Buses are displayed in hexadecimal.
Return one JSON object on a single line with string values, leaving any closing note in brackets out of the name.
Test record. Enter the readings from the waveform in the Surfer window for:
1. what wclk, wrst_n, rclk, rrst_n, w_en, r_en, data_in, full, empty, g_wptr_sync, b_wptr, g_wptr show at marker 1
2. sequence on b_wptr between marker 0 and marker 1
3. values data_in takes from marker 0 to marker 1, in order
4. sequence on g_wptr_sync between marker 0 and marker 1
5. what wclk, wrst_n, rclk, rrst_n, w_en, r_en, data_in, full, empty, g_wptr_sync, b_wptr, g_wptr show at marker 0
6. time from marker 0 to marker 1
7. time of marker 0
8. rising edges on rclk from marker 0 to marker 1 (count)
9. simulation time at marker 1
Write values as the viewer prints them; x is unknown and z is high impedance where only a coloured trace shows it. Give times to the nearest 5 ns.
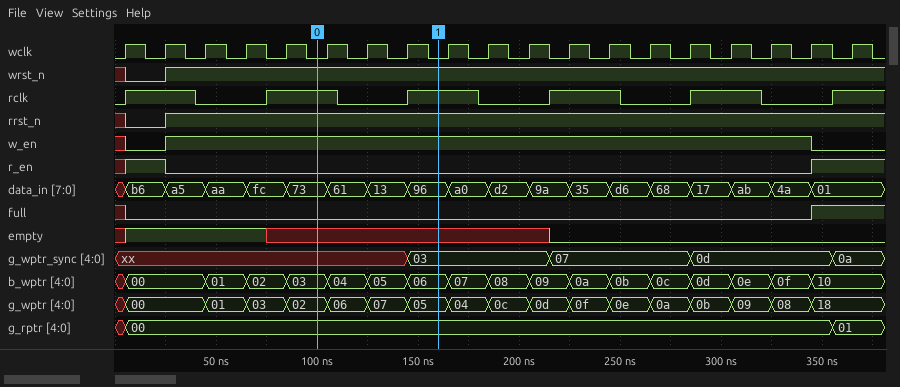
{"what wclk, wrst_n, rclk, rrst_n, w_en, r_en, data_in, full, empty, g_wptr_sync, b_wptr, g_wptr show at marker 1": "wclk=0, wrst_n=1, rclk=1, rrst_n=1, w_en=1, r_en=0, data_in=96, full=0, empty=x, g_wptr_sync=03, b_wptr=06, g_wptr=05", "sequence on b_wptr between marker 0 and marker 1": "03, 04, 05, 06", "values data_in takes from marker 0 to marker 1, in order": "73, 61, 13, 96", "sequence on g_wptr_sync between marker 0 and marker 1": "xx, 03", "what wclk, wrst_n, rclk, rrst_n, w_en, r_en, data_in, full, empty, g_wptr_sync, b_wptr, g_wptr show at marker 0": "wclk=0, wrst_n=1, rclk=1, rrst_n=1, w_en=1, r_en=0, data_in=73, full=0, empty=x, g_wptr_sync=xx, b_wptr=03, g_wptr=02", "time from marker 0 to marker 1": "60 ns", "time of marker 0": "100 ns", "rising edges on rclk from marker 0 to marker 1": "1", "simulation time at marker 1": "160 ns"}
